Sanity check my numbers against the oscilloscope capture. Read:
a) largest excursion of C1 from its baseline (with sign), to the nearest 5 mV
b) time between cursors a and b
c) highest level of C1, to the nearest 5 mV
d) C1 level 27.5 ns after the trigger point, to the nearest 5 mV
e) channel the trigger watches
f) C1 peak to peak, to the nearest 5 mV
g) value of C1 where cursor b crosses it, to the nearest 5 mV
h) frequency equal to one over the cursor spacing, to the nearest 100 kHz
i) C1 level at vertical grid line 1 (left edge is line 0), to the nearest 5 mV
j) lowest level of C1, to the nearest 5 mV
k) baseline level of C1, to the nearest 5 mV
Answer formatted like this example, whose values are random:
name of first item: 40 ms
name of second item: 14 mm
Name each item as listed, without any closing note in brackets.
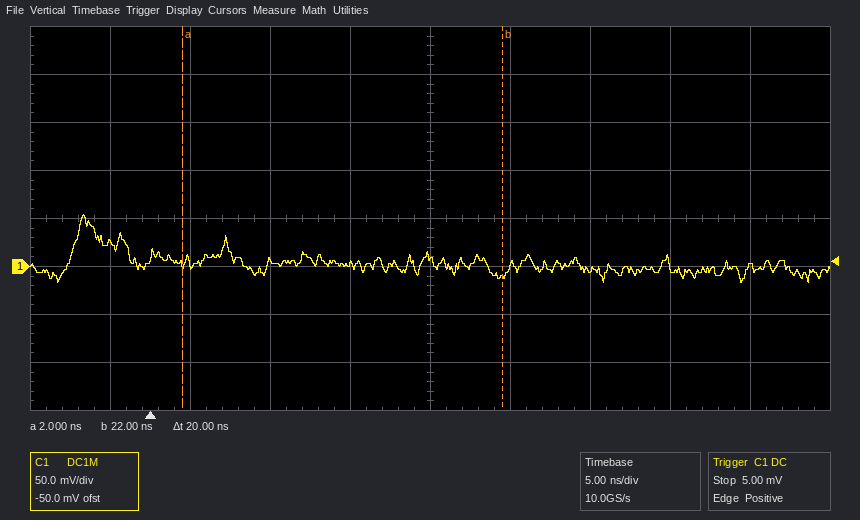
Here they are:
largest excursion of C1 from its baseline (with sign), to the nearest 5 mV: +55 mV
time between cursors a and b: 20 ns
highest level of C1, to the nearest 5 mV: 55 mV
C1 level 27.5 ns after the trigger point, to the nearest 5 mV: -5 mV
channel the trigger watches: C1
C1 peak to peak, to the nearest 5 mV: 70 mV
value of C1 where cursor b crosses it, to the nearest 5 mV: -10 mV
frequency equal to one over the cursor spacing, to the nearest 100 kHz: 50.0 MHz
C1 level at vertical grid line 1 (left edge is line 0), to the nearest 5 mV: 25 mV
lowest level of C1, to the nearest 5 mV: -15 mV
baseline level of C1, to the nearest 5 mV: 0 mV
